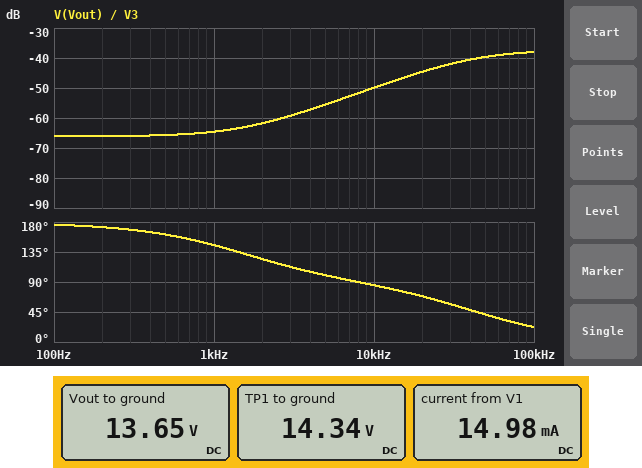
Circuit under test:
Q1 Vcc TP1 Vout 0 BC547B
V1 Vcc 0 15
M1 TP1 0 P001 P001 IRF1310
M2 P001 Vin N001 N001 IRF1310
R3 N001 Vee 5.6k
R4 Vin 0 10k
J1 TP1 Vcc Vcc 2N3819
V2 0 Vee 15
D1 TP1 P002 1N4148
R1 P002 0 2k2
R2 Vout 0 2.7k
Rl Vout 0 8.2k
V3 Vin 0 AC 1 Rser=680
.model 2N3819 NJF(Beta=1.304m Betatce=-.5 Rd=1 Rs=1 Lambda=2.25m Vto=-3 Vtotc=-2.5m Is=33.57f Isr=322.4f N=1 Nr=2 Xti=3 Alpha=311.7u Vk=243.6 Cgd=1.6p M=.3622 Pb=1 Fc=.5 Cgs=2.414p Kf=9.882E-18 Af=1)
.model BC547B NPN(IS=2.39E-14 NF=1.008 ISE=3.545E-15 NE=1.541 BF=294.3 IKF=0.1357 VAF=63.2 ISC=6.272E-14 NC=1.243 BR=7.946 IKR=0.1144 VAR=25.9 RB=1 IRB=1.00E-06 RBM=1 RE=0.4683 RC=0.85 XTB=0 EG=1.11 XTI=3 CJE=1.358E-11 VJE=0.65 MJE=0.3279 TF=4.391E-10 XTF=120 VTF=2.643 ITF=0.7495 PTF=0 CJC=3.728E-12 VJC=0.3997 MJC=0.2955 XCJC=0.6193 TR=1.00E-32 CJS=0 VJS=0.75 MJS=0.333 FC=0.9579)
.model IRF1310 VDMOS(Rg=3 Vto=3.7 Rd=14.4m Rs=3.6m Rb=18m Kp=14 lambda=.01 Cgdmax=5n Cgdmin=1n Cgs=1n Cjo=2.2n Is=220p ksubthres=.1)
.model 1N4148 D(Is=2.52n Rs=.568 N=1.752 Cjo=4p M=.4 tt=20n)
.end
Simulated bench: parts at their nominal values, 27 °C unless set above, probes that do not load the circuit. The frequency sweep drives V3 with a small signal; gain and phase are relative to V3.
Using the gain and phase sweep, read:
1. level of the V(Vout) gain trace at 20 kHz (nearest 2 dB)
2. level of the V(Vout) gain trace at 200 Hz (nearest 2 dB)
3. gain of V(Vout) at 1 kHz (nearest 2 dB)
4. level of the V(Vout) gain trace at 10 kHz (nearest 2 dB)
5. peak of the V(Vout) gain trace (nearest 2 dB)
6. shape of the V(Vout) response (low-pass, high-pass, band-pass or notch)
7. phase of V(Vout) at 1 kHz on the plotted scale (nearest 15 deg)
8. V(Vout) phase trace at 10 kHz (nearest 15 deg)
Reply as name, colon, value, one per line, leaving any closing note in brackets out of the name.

level of the V(Vout) gain trace at 20 kHz: -44 dB
level of the V(Vout) gain trace at 200 Hz: -66 dB
gain of V(Vout) at 1 kHz: -64 dB
level of the V(Vout) gain trace at 10 kHz: -50 dB
peak of the V(Vout) gain trace: -38 dB
shape of the V(Vout) response: high-pass
phase of V(Vout) at 1 kHz on the plotted scale: 150 deg
V(Vout) phase trace at 10 kHz: 90 deg
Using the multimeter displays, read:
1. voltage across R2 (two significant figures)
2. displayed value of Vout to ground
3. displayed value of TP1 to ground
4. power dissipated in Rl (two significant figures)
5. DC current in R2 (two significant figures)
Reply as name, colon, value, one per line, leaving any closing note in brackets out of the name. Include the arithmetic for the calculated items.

voltage across R2: 13.65 V = 14 V
displayed value of Vout to ground: 13.65 V
displayed value of TP1 to ground: 14.34 V
power dissipated in Rl: (13.65 V)^2 / 8.2 kΩ = 23 mW
DC current in R2: (13.65 V) / 2.7 kΩ = 5.1 mA
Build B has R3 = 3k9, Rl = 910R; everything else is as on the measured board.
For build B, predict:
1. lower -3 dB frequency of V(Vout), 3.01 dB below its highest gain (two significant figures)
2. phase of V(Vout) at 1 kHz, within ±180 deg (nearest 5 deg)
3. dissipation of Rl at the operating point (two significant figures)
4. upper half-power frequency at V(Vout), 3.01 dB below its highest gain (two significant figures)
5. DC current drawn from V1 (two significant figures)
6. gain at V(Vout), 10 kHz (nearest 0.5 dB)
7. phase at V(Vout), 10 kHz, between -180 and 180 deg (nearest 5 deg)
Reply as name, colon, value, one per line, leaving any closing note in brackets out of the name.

lower -3 dB frequency of V(Vout), 3.01 dB below its highest gain: 42 kHz
phase of V(Vout) at 1 kHz, within ±180 deg: 155 deg
dissipation of Rl at the operating point: 200 mW
upper half-power frequency at V(Vout), 3.01 dB below its highest gain: 5.1 MHz
DC current drawn from V1: 29 mA
gain at V(Vout), 10 kHz: -52.0 dB
phase at V(Vout), 10 kHz, between -180 and 180 deg: 90 deg
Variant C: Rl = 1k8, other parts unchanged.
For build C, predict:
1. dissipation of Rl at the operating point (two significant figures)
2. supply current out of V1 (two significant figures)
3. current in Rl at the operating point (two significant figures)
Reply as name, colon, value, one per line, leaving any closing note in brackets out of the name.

dissipation of Rl at the operating point: 100 mW
supply current out of V1: 21 mA
current in Rl at the operating point: 7.6 mA
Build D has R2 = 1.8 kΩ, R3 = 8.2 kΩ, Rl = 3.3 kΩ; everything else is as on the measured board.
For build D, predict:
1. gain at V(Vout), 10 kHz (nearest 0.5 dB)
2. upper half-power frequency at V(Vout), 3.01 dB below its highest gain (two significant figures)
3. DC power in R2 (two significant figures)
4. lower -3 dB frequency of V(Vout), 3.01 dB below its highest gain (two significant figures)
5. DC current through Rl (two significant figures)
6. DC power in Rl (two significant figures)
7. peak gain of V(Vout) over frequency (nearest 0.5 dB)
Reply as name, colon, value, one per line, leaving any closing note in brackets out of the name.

gain at V(Vout), 10 kHz: -48.5 dB
upper half-power frequency at V(Vout), 3.01 dB below its highest gain: 3.0 MHz
DC power in R2: 100 mW
lower -3 dB frequency of V(Vout), 3.01 dB below its highest gain: 40 kHz
DC current through Rl: 4.1 mA
DC power in Rl: 56 mW
peak gain of V(Vout) over frequency: -36.0 dB
